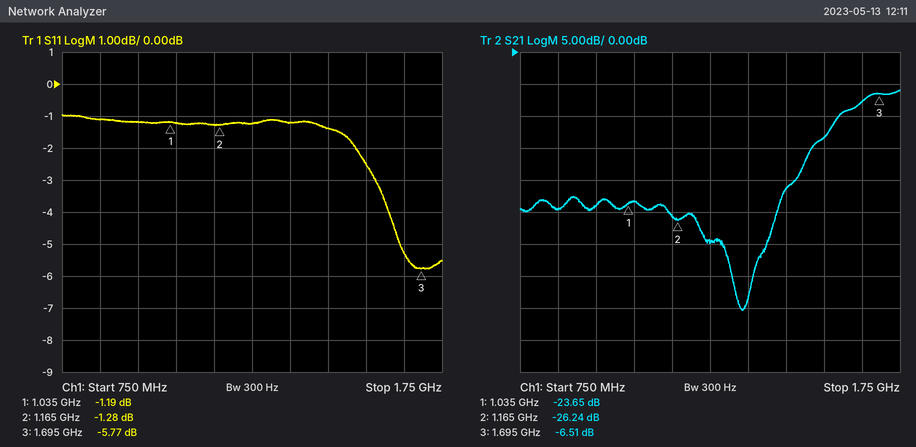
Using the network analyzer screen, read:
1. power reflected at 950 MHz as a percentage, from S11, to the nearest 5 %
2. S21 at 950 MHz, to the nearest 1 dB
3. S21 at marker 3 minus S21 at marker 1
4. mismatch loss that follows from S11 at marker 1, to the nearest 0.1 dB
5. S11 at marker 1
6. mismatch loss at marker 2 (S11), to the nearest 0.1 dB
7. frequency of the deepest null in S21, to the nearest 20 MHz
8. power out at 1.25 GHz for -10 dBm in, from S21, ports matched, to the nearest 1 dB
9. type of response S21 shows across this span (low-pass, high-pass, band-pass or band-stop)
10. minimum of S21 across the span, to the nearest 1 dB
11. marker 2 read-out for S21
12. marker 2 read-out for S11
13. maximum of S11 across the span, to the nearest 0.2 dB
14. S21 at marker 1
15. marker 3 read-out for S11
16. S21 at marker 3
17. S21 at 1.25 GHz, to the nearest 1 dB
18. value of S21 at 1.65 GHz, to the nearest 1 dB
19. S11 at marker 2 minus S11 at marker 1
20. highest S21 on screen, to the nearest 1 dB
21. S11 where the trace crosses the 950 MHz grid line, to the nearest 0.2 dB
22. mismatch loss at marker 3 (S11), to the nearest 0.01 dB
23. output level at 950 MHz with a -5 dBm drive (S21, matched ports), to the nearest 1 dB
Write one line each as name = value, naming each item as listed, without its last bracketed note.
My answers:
power reflected at 950 MHz as a percentage, from S11, to the nearest 5 % = 75 %
S21 at 950 MHz, to the nearest 1 dB = -24 dB
S21 at marker 3 minus S21 at marker 1 = 17.14 dB
mismatch loss that follows from S11 at marker 1, to the nearest 0.1 dB = 6.2 dB
S11 at marker 1 = -1.19 dB
mismatch loss at marker 2 (S11), to the nearest 0.1 dB = 5.9 dB
frequency of the deepest null in S21, to the nearest 20 MHz = 1.34 GHz
power out at 1.25 GHz for -10 dBm in, from S21, ports matched, to the nearest 1 dB = -40 dBm
type of response S21 shows across this span = high-pass
minimum of S21 across the span, to the nearest 1 dB = -40 dB
marker 2 read-out for S21 = -26.24 dB
marker 2 read-out for S11 = -1.28 dB
maximum of S11 across the span, to the nearest 0.2 dB = -1.0 dB
S21 at marker 1 = -23.65 dB
marker 3 read-out for S11 = -5.77 dB
S21 at marker 3 = -6.51 dB
S21 at 1.25 GHz, to the nearest 1 dB = -30 dB
value of S21 at 1.65 GHz, to the nearest 1 dB = -8 dB
S11 at marker 2 minus S11 at marker 1 = -0.09 dB
highest S21 on screen, to the nearest 1 dB = -6 dB
S11 where the trace crosses the 950 MHz grid line, to the nearest 0.2 dB = -1.2 dB
mismatch loss at marker 3 (S11), to the nearest 0.01 dB = 1.34 dB
output level at 950 MHz with a -5 dBm drive (S21, matched ports), to the nearest 1 dB = -29 dBm
